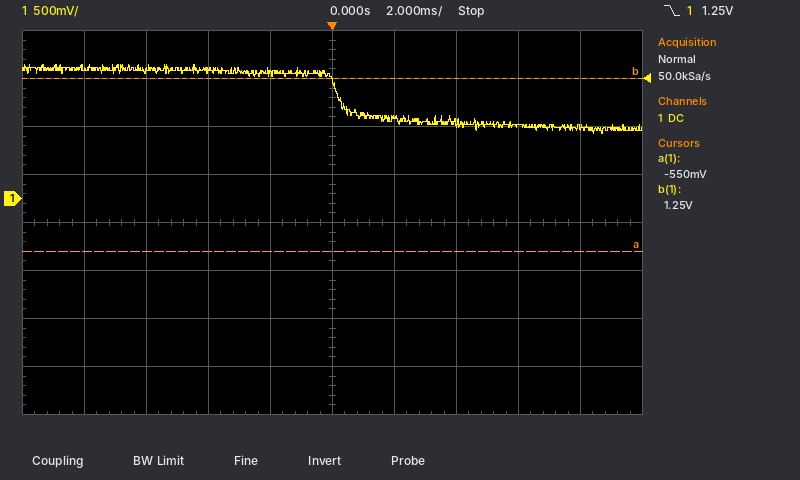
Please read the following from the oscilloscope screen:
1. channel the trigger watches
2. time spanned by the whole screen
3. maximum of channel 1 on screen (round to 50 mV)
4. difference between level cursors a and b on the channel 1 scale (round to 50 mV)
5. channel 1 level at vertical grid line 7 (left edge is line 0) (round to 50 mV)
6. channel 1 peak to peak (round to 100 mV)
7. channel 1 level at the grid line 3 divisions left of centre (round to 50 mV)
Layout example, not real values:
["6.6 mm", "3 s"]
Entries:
["channel 1", "20 ms", "1.40 V", "1.80 V", "800 mV", "700 mV", "1.35 V"]
